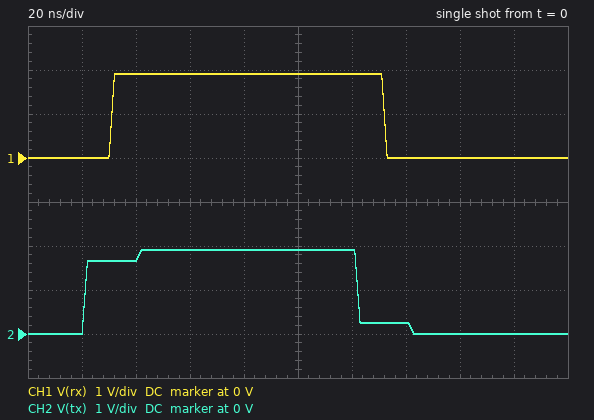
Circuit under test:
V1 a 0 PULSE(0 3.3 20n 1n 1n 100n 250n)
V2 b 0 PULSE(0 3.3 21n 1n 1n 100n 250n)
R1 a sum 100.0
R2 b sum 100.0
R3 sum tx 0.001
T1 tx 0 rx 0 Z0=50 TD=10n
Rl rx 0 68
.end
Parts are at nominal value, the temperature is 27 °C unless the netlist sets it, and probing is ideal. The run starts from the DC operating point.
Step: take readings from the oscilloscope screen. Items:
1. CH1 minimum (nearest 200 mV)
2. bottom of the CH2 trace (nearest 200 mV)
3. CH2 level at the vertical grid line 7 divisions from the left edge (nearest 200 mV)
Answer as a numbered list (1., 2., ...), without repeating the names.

1. 0 V
2. 0 V
3. 200 mV
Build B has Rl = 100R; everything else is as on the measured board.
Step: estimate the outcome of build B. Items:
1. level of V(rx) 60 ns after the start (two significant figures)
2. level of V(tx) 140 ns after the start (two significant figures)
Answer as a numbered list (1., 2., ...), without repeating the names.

1. 2.2 V
2. 550 mV
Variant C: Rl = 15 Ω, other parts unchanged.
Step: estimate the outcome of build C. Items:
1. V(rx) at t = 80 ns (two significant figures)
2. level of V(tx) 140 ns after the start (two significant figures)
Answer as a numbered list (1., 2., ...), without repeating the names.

1. 760 mV
2. -890 mV
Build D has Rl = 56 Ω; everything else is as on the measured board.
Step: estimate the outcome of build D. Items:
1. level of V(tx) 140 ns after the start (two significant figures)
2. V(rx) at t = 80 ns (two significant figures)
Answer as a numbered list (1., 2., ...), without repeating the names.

1. 93 mV
2. 1.7 V
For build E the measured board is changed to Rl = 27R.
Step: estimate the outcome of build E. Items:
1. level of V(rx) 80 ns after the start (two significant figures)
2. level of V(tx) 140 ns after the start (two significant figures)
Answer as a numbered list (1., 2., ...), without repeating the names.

1. 1.2 V
2. -490 mV
